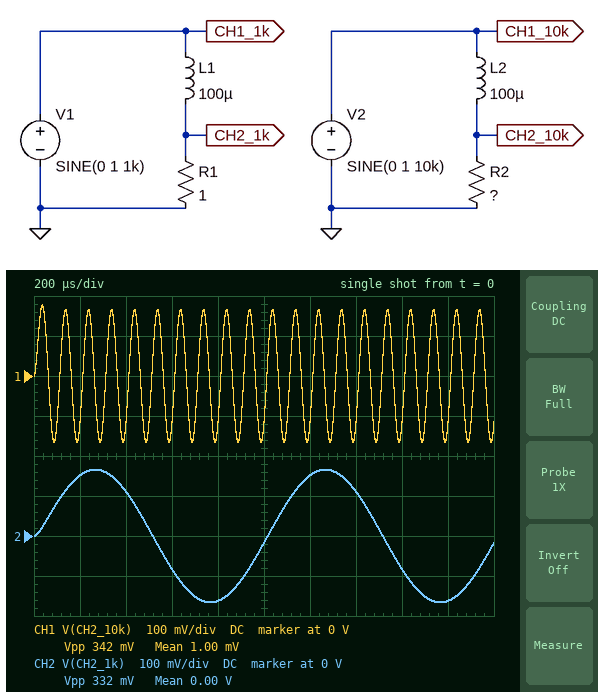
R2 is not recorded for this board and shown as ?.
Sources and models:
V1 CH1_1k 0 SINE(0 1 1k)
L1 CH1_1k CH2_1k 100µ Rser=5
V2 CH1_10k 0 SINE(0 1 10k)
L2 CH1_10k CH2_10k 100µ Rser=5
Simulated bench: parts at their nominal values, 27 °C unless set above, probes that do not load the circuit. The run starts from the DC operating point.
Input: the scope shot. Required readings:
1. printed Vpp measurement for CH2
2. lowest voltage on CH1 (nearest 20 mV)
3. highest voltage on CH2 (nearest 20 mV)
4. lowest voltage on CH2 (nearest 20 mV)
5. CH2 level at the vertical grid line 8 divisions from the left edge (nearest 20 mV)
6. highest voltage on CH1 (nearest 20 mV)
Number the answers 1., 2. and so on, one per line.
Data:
1. 332 mV
2. -160 mV
3. 160 mV
4. -160 mV
5. -80 mV
6. 180 mV
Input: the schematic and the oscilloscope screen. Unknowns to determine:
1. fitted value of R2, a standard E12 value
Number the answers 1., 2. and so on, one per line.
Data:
1. 1.5 Ω
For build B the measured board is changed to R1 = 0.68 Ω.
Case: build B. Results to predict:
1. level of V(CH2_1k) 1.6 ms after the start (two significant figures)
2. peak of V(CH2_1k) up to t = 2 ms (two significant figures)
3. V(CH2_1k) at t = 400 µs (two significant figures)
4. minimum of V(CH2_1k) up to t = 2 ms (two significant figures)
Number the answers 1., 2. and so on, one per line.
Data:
1. -59 mV
2. 120 mV
3. 80 mV
4. -120 mV
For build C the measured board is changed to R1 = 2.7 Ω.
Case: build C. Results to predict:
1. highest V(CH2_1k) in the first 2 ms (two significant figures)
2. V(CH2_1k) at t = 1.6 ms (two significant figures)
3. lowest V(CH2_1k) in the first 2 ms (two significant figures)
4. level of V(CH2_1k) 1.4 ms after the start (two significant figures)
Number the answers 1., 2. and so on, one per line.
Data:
1. 350 mV
2. -180 mV
3. -350 mV
4. 230 mV
